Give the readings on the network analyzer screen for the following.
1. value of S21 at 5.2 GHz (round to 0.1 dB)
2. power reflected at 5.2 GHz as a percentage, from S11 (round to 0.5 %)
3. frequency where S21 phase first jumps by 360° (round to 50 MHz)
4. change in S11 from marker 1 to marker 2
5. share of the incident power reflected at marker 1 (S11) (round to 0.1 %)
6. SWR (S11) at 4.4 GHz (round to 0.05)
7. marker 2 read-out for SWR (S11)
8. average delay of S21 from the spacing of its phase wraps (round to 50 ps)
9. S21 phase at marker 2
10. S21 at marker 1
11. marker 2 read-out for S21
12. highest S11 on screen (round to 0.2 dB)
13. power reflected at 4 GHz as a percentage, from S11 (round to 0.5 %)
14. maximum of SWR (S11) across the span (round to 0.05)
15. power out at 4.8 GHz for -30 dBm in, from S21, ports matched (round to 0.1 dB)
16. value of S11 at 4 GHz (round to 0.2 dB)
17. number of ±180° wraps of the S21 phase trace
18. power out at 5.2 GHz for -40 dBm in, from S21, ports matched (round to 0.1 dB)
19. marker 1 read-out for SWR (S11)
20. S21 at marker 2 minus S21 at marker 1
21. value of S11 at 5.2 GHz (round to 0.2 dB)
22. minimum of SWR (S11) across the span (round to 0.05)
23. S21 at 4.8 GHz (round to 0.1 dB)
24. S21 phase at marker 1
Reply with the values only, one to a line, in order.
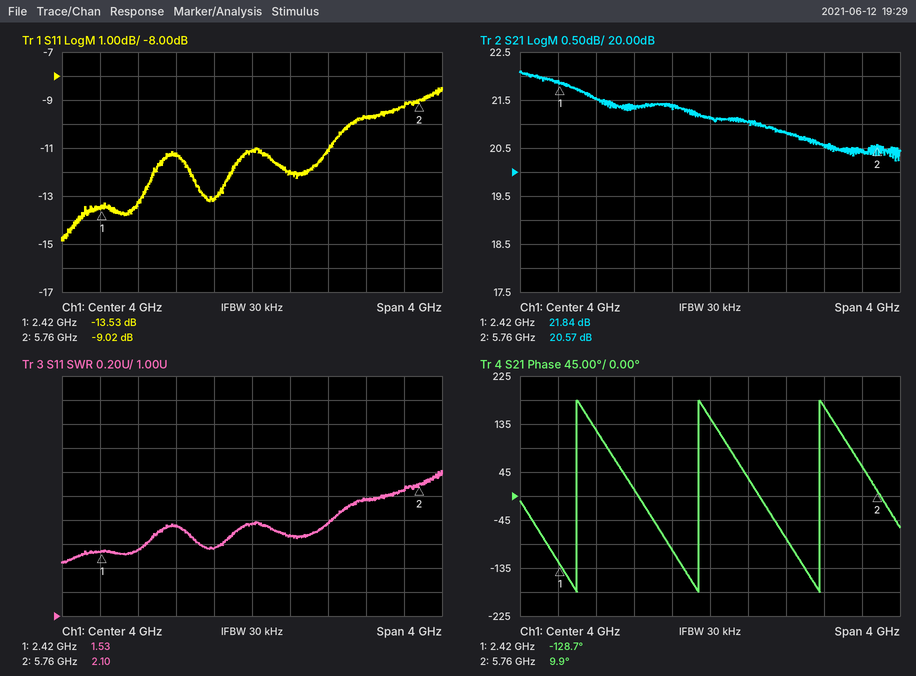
20.6 dB
10.5 %
2.60 GHz
4.51 dB
4.4 %
1.65
2.10
800 ps
9.9°
21.84 dB
20.57 dB
-8.4 dB
7.5 %
2.20
-9.2 dBm
-11.2 dB
3
-19.4 dBm
1.53
-1.27 dB
-9.8 dB
1.45
20.8 dB
-128.7°
